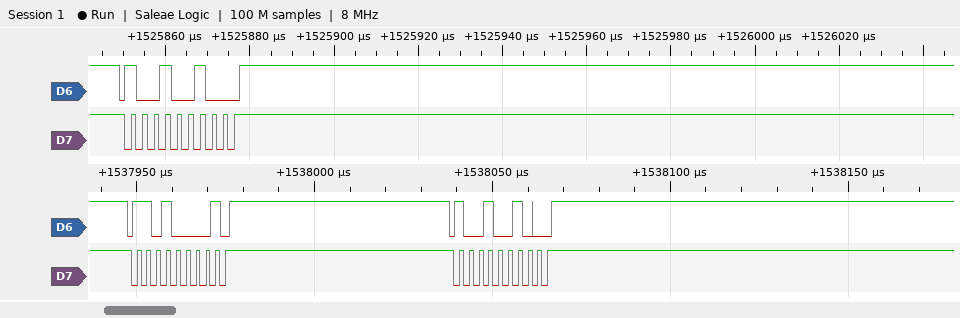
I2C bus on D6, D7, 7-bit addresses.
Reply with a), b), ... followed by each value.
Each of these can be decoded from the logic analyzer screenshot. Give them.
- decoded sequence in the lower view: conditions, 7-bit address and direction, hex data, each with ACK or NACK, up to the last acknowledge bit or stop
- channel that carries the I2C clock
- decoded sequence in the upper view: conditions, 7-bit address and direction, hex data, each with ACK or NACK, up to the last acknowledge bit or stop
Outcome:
a) start, address 68 write NACK, stop, start, address 49 write ACK, stop
b) D7
c) start, address 49 write ACK, stop
